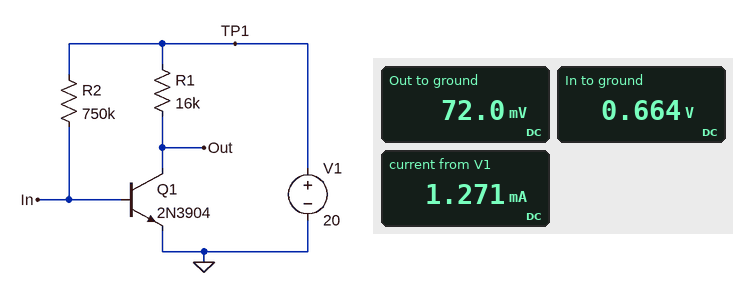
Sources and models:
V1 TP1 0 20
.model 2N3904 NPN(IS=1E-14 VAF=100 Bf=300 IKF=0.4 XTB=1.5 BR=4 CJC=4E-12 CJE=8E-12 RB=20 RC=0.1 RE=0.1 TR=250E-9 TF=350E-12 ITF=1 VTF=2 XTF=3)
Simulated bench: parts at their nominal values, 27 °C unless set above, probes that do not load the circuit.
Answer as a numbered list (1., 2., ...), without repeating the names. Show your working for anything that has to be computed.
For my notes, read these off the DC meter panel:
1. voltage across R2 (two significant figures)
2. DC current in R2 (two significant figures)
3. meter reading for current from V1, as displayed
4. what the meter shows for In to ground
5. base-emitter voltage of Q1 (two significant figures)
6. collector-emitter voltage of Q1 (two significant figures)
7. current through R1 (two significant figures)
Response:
1. 20 V - 664 mV = 19 V
2. (20 V - 664 mV) / 750 kΩ = 26 µA
3. 1.271 mA
4. 0.664 V
5. 664 mV = 660 mV
6. 72 mV = 72 mV
7. (20 V - 72 mV) / 16 kΩ = 1.2 mA
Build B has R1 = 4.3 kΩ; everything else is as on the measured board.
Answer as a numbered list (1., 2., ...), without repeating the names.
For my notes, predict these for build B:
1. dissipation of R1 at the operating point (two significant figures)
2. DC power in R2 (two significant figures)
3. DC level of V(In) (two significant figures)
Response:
1. 92 mW
2. 500 µW
3. 700 mV
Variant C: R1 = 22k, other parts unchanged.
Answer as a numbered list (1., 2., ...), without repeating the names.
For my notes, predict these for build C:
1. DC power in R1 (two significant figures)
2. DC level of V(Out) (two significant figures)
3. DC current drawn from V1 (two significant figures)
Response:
1. 18 mW
2. 63 mV
3. 930 µA
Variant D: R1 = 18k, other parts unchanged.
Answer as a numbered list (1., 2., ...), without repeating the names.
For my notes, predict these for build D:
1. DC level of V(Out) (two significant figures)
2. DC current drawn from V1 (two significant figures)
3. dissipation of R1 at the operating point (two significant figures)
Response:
1. 69 mV
2. 1.1 mA
3. 22 mW
